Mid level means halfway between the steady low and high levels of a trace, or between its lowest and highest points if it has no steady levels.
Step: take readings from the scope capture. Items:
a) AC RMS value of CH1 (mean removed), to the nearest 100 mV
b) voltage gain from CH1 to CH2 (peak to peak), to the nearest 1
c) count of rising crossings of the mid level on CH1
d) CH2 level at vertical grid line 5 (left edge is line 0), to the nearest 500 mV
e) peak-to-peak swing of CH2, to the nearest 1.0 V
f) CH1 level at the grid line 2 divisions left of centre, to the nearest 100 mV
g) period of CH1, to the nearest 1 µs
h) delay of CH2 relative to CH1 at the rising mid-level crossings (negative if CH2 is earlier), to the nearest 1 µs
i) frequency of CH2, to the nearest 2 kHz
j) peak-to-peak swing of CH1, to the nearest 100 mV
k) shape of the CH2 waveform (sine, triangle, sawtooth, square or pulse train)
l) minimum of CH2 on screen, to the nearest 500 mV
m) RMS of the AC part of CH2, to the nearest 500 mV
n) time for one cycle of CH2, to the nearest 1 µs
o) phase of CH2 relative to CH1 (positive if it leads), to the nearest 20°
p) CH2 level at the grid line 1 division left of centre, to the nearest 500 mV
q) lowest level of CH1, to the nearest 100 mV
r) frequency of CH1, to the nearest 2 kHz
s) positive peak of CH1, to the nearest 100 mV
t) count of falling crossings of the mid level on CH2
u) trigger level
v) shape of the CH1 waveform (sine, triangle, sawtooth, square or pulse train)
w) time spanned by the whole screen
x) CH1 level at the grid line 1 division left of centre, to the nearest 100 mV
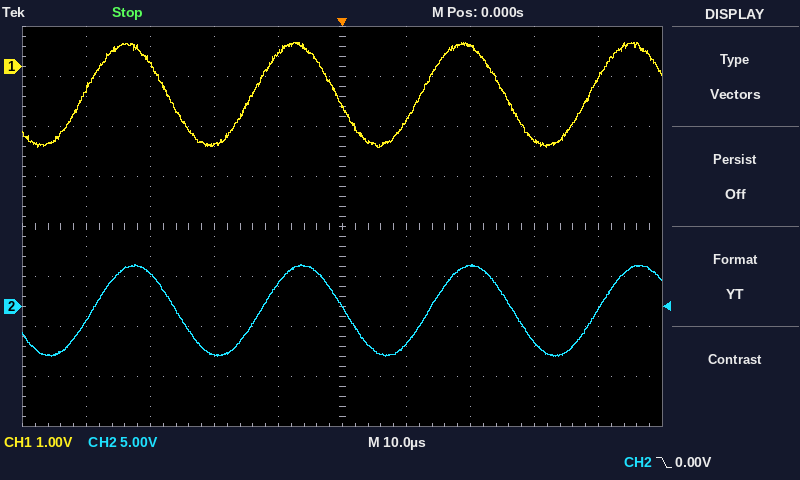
700 mV
4
4
0.0 V
9.0 V
-1.6 V
26 µs
+1 µs
38 kHz
2.1 V
sine
-5.0 V
3.0 V
26 µs
-20°
2.5 V
-1.6 V
38 kHz
500 mV
3
0.00 V
sine
100 µs
300 mV
